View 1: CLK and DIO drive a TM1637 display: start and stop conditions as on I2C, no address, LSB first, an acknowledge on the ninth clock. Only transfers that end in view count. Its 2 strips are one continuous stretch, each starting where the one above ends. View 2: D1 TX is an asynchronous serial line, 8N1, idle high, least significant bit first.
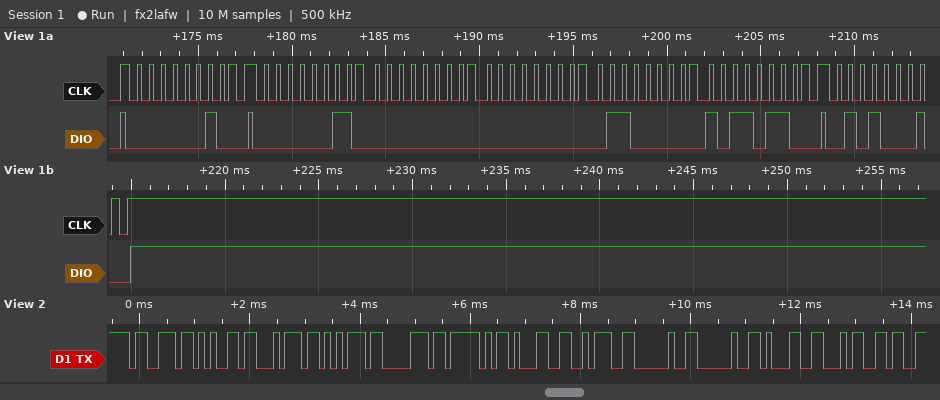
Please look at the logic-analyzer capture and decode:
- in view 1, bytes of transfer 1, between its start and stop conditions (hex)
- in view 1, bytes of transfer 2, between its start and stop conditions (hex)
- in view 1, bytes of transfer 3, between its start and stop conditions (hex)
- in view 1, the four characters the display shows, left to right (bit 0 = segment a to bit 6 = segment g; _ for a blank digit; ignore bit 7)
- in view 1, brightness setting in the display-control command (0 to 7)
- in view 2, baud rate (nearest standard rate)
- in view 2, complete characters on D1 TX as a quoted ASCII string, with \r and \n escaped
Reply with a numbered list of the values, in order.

1. 40
2. C0 00 00 06 6D
3. 8A
4. __15
5. 2
6. 9600 baud
7. "setup_1:  14"
